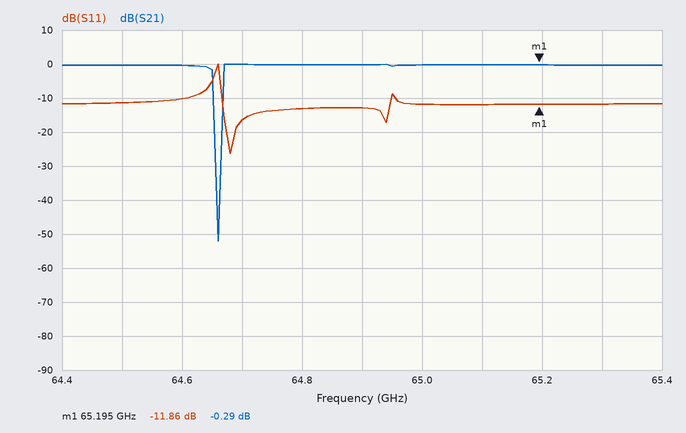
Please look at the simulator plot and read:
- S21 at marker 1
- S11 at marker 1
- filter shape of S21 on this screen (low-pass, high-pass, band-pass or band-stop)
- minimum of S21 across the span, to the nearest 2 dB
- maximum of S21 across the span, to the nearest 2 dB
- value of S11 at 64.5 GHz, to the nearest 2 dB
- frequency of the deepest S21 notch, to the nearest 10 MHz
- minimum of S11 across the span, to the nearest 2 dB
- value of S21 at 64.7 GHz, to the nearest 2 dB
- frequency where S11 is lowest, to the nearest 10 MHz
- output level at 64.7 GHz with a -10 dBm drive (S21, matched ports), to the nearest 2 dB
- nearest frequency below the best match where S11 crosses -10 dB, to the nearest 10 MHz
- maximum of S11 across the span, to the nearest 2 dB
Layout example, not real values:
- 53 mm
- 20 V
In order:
- -0.29 dB
- -11.86 dB
- band-stop
- -52 dB
- 0 dB
- -12 dB
- 64.66 GHz
- -26 dB
- 0 dB
- 64.68 GHz
- -10 dBm
- 64.67 GHz
- 0 dB
